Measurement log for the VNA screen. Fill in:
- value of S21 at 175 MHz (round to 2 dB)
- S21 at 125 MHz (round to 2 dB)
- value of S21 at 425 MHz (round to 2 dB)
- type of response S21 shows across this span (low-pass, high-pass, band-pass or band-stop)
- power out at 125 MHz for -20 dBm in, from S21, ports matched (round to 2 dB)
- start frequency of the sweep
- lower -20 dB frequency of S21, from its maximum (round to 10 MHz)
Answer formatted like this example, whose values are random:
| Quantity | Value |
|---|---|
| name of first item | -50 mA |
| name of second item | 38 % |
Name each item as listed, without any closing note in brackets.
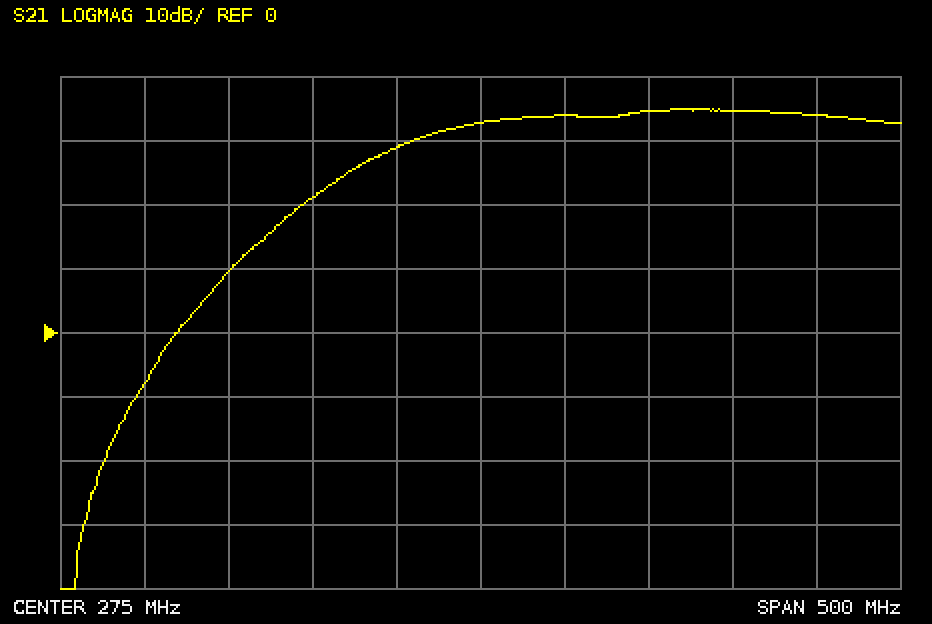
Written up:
| Quantity | Value |
|---|---|
| value of S21 at 175 MHz | 22 dB |
| S21 at 125 MHz | 10 dB |
| value of S21 at 425 MHz | 34 dB |
| type of response S21 shows across this span | high-pass |
| power out at 125 MHz for -20 dBm in, from S21, ports matched | -10 dBm |
| start frequency of the sweep | 25 MHz |
| lower -20 dB frequency of S21, from its maximum | 150 MHz |
